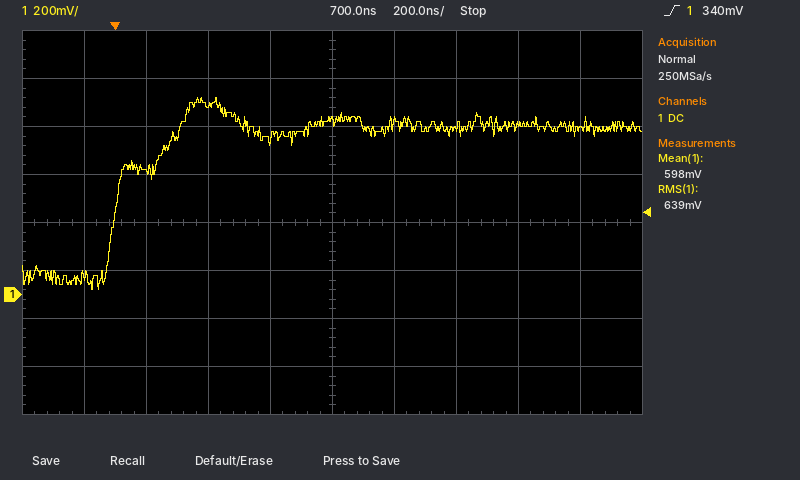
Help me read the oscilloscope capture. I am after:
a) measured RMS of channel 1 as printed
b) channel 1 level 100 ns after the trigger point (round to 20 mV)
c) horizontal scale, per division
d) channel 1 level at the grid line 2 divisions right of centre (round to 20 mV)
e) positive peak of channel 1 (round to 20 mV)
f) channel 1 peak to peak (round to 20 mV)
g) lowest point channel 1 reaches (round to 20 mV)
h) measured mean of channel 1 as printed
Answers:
639 mV
520 mV
200 ns
700 mV
820 mV
800 mV
20 mV
598 mV
